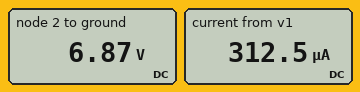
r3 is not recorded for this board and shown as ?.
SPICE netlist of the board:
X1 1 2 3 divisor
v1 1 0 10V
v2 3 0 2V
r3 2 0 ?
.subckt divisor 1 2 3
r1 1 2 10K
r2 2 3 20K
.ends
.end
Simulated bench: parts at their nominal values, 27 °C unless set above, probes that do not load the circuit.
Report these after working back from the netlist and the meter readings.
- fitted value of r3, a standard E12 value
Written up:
100 kΩ
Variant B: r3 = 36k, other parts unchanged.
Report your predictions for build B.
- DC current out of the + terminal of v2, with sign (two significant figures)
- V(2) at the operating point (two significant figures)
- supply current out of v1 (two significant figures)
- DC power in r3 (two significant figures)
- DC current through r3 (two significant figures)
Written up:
-210 µA
6.2 V
380 µA
1.1 mW
170 µA
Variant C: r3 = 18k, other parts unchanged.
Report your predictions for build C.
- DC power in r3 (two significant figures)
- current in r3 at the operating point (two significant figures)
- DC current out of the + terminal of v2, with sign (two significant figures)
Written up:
1.6 mW
300 µA
-170 µA
